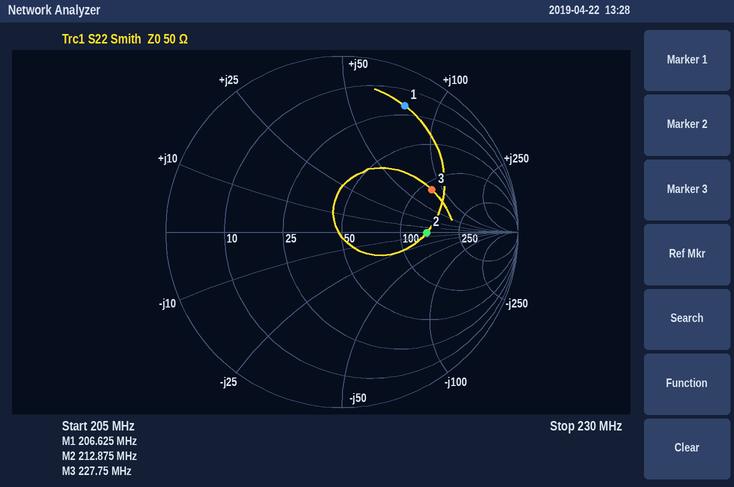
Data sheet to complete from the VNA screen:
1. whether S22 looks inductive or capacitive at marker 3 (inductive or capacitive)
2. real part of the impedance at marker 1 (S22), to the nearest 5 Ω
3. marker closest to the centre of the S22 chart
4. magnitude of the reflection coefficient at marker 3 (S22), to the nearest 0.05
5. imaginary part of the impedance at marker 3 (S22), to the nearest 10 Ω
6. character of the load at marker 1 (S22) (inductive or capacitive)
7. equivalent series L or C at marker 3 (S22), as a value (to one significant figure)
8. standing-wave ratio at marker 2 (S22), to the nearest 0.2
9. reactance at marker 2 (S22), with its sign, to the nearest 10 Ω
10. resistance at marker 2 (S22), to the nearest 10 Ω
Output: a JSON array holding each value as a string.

["inductive", "20 Ω", "marker 2", "0.55", "+80 Ω", "inductive", "60 nH", "2.8", "0 Ω", "140 Ω"]
